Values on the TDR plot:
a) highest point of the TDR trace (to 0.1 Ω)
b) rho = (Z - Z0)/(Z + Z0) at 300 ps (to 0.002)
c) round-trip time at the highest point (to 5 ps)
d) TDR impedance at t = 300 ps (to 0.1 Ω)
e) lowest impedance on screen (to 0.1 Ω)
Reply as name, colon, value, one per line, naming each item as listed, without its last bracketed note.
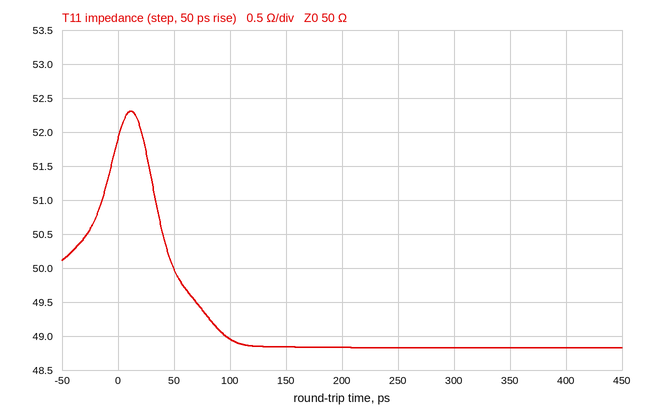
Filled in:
highest point of the TDR trace: 52.3 Ω
rho = (Z - Z0)/(Z + Z0) at 300 ps: -0.012
round-trip time at the highest point: 10 ps
TDR impedance at t = 300 ps: 48.8 Ω
lowest impedance on screen: 48.8 Ω
